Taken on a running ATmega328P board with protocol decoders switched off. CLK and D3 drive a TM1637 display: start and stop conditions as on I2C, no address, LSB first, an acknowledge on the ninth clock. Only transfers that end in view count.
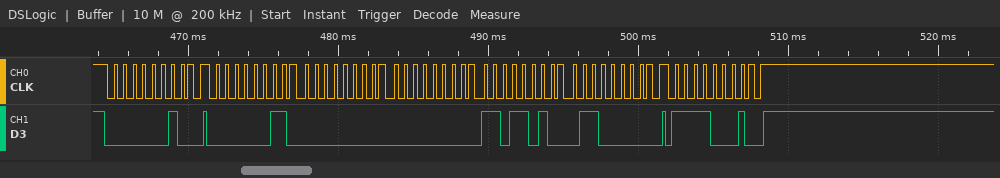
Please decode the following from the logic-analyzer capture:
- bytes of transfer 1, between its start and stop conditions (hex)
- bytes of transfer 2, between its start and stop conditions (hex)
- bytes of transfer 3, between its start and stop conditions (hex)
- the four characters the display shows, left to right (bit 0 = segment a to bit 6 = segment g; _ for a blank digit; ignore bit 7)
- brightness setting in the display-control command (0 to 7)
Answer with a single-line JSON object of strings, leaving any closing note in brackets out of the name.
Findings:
{"bytes of transfer 1, between its start and stop conditions": "40", "bytes of transfer 2, between its start and stop conditions": "C0 00 00 5B 06", "bytes of transfer 3, between its start and stop conditions": "8F", "the four characters the display shows, left to right": "__21", "brightness setting in the display-control command": "7"}
